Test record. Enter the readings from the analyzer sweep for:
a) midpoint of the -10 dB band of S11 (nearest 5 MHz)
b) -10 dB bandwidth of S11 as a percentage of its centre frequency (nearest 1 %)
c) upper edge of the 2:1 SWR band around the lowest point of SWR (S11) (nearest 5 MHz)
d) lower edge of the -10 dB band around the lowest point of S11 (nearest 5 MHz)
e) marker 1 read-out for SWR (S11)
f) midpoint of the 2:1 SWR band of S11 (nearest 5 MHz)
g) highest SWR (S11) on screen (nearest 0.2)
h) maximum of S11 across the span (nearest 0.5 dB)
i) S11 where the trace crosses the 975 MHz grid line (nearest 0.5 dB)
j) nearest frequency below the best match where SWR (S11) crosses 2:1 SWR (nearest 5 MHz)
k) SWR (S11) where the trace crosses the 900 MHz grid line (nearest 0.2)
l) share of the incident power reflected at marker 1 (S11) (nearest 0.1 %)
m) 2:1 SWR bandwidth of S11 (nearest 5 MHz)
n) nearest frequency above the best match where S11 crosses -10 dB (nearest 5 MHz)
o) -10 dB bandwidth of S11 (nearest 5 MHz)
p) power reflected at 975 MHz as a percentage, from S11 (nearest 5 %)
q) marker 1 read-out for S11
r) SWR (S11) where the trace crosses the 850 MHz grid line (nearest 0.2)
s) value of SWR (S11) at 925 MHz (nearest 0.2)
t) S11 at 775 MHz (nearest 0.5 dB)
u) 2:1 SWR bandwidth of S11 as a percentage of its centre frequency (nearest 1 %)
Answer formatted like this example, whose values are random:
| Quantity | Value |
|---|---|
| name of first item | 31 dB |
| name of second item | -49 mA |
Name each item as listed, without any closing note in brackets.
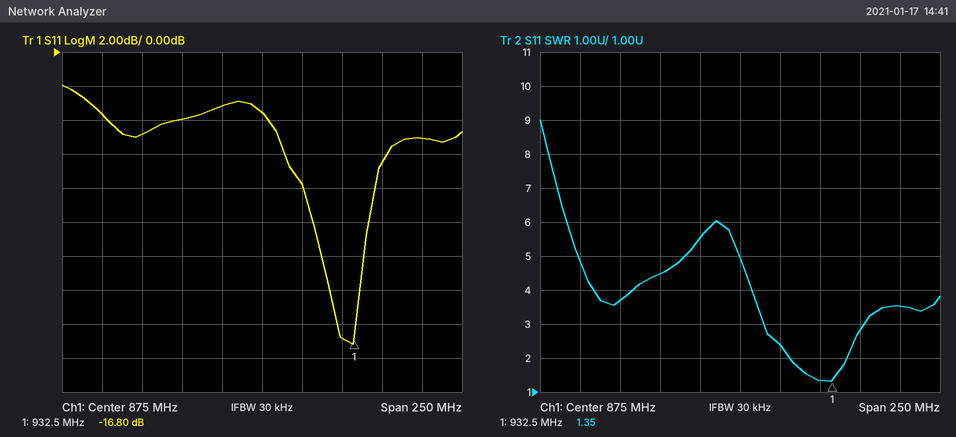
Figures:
| Quantity | Value |
|---|---|
| midpoint of the -10 dB band of S11 | 925 MHz |
| -10 dB bandwidth of S11 as a percentage of its centre frequency | 4 % |
| upper edge of the 2:1 SWR band around the lowest point of SWR (S11) | 940 MHz |
| lower edge of the -10 dB band around the lowest point of S11 | 905 MHz |
| marker 1 read-out for SWR | 1.35 |
| midpoint of the 2:1 SWR band of S11 | 925 MHz |
| highest SWR (S11) on screen | 9.0 |
| maximum of S11 across the span | -2.0 dB |
| S11 where the trace crosses the 975 MHz grid line | -5.0 dB |
| nearest frequency below the best match where SWR (S11) crosses 2:1 SWR | 905 MHz |
| SWR (S11) where the trace crosses the 900 MHz grid line | 2.4 |
| share of the incident power reflected at marker 1 (S11) | 2.1 % |
| 2:1 SWR bandwidth of S11 | 35 MHz |
| nearest frequency above the best match where S11 crosses -10 dB | 940 MHz |
| -10 dB bandwidth of S11 | 35 MHz |
| power reflected at 975 MHz as a percentage, from S11 | 30 % |
| marker 1 read-out for S11 | -16.80 dB |
| SWR (S11) where the trace crosses the 850 MHz grid line | 5.6 |
| value of SWR (S11) at 925 MHz | 1.4 |
| S11 at 775 MHz | -3.5 dB |
| 2:1 SWR bandwidth of S11 as a percentage of its centre frequency | 4 % |
